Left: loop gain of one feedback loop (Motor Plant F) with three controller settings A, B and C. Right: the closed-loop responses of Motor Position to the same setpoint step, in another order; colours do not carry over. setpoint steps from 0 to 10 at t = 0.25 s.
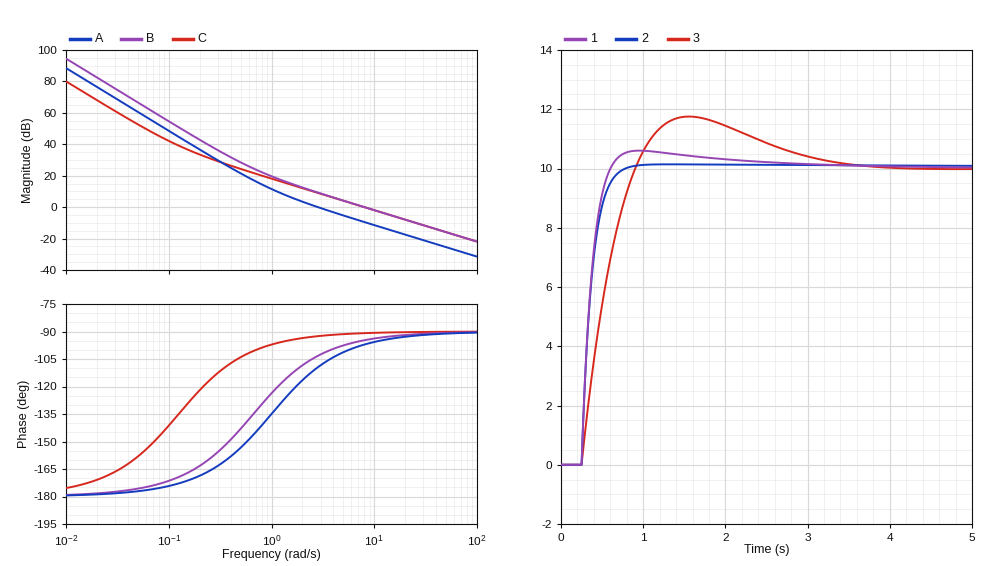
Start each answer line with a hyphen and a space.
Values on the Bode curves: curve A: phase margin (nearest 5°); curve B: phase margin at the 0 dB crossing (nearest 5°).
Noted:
- 70°
- 85°
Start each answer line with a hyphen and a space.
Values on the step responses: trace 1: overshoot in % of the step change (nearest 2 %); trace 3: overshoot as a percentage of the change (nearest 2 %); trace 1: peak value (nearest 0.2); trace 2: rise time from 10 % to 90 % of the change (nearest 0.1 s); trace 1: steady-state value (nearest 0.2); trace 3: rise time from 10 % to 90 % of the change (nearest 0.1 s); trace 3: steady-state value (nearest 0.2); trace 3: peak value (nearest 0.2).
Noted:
- 6 %
- 18 %
- 10.6
- 0.3 s
- 10.0
- 0.5 s
- 10.0
- 11.8
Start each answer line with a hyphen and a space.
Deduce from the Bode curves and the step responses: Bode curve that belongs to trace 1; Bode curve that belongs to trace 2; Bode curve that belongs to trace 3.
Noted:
- B
- C
- A
